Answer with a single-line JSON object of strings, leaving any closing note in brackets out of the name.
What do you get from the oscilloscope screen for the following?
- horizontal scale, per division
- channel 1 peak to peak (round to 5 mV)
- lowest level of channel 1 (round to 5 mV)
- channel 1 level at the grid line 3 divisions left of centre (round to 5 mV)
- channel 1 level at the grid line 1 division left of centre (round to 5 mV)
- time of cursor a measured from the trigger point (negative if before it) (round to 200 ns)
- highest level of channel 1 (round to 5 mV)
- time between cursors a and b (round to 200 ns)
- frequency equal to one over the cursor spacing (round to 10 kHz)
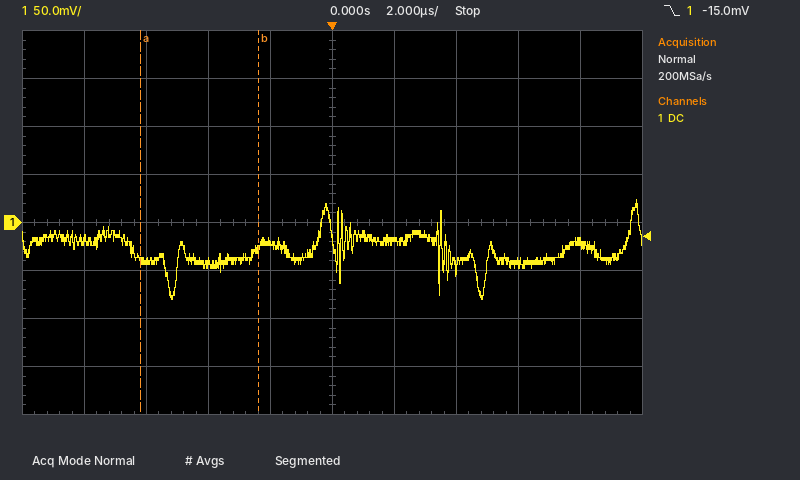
{"horizontal scale, per division": "2 µs", "channel 1 peak to peak": "105 mV", "lowest level of channel 1": "-80 mV", "channel 1 level at the grid line 3 divisions left of centre": "-40 mV", "channel 1 level at the grid line 1 division left of centre": "-20 mV", "time of cursor a measured from the trigger point (negative if before it)": "-6.2 µs", "highest level of channel 1": "25 mV", "time between cursors a and b": "3.8 µs", "frequency equal to one over the cursor spacing": "260 kHz"}
